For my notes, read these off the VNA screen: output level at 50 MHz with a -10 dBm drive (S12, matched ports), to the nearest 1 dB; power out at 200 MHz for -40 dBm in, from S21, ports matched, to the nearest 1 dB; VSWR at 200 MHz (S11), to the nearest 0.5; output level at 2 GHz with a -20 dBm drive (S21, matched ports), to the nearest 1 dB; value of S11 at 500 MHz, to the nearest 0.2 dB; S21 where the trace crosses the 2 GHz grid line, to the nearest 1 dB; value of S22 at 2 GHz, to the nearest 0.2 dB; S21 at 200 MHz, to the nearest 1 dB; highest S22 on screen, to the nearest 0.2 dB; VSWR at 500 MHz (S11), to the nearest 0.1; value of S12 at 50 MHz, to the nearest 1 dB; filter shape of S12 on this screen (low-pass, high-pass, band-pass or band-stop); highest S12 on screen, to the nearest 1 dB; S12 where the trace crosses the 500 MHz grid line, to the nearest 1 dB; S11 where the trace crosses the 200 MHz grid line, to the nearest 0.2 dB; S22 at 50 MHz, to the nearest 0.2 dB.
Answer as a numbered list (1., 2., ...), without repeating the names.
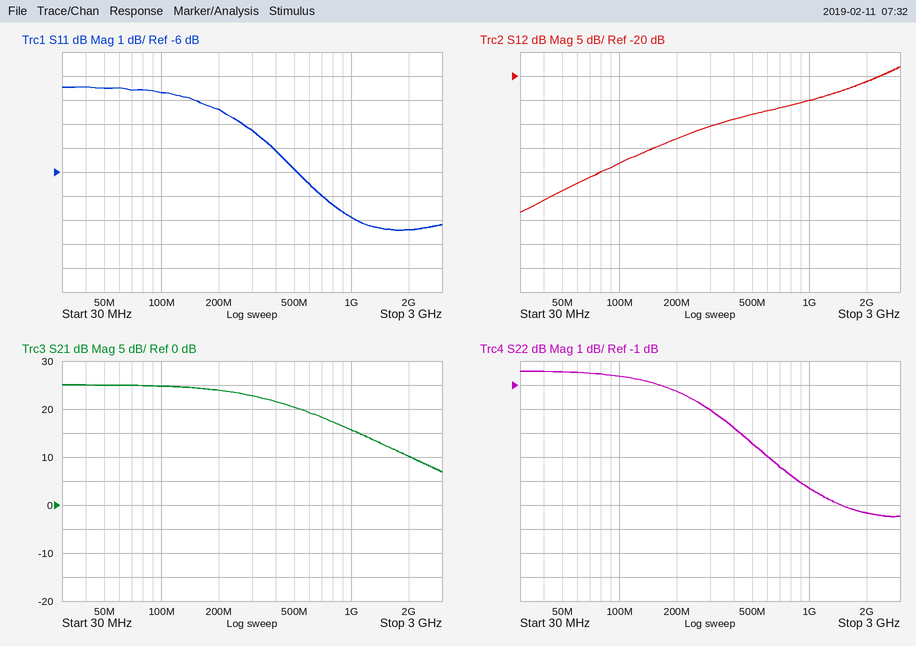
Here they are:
1. -54 dBm
2. -16 dBm
3. 5.0
4. -10 dBm
5. -5.8 dB
6. 10 dB
7. -6.4 dB
8. 24 dB
9. -0.4 dB
10. 3.1
11. -44 dB
12. high-pass
13. -18 dB
14. -28 dB
15. -3.4 dB
16. -0.4 dB
